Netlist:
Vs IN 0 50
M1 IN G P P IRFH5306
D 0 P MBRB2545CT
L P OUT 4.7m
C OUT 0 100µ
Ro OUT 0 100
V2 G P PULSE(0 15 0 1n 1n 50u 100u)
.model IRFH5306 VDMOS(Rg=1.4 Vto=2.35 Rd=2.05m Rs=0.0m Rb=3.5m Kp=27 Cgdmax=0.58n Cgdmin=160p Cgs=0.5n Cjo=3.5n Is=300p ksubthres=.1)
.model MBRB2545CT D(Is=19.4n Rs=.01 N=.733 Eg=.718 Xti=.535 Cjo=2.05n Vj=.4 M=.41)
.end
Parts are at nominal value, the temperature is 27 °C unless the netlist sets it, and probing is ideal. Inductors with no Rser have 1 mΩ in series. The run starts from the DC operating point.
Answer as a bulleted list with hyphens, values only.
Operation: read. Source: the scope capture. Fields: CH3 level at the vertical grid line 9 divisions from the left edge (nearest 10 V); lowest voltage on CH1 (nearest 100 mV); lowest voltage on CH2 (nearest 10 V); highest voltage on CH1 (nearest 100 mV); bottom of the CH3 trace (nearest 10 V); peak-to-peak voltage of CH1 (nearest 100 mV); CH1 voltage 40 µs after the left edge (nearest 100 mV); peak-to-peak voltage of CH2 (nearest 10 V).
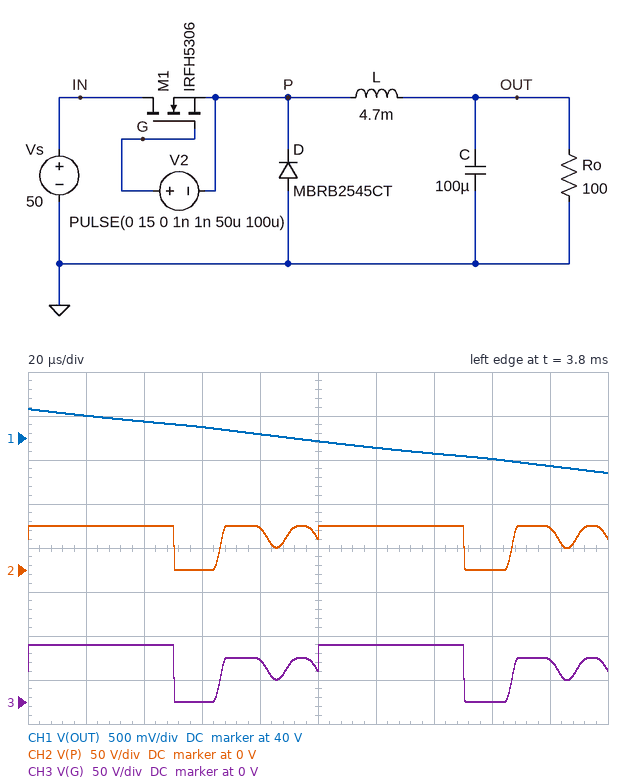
- 50 V
- 39.6 V
- 0 V
- 40.3 V
- 0 V
- 700 mV
- 40.2 V
- 50 V
